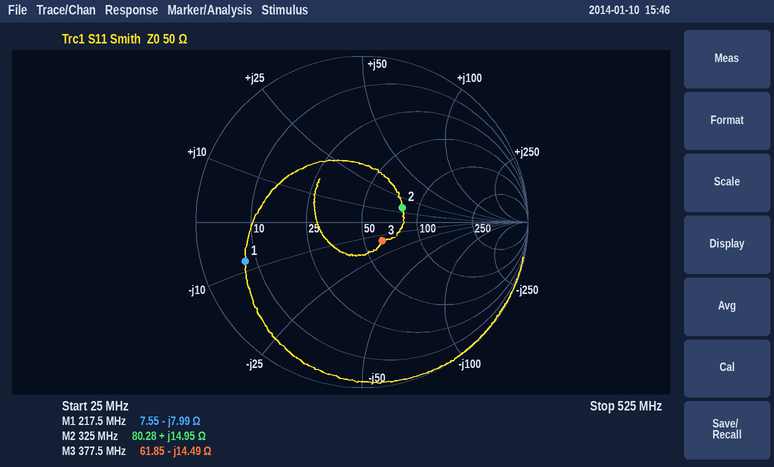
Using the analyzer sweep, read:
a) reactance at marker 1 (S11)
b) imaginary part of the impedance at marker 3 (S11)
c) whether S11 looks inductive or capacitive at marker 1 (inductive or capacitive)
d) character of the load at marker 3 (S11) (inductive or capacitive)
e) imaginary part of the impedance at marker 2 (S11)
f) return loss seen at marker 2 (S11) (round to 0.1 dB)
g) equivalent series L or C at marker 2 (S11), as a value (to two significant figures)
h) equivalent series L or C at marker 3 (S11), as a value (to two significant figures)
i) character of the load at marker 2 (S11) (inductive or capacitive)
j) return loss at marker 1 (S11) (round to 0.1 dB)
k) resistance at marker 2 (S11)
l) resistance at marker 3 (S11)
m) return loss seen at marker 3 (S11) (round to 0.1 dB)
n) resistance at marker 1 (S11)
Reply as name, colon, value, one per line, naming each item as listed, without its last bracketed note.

reactance at marker 1: -7.99 Ω
imaginary part of the impedance at marker 3: -14.49 Ω
whether S11 looks inductive or capacitive at marker 1: capacitive
character of the load at marker 3 (S11): capacitive
imaginary part of the impedance at marker 2: +14.95 Ω
return loss seen at marker 2 (S11): 11.8 dB
equivalent series L or C at marker 2 (S11), as a value: 7.3 nH
equivalent series L or C at marker 3 (S11), as a value: 29 pF
character of the load at marker 2 (S11): inductive
return loss at marker 1 (S11): 2.6 dB
resistance at marker 2: 80.28 Ω
resistance at marker 3: 61.85 Ω
return loss seen at marker 3 (S11): 15.6 dB
resistance at marker 1: 7.55 Ω
